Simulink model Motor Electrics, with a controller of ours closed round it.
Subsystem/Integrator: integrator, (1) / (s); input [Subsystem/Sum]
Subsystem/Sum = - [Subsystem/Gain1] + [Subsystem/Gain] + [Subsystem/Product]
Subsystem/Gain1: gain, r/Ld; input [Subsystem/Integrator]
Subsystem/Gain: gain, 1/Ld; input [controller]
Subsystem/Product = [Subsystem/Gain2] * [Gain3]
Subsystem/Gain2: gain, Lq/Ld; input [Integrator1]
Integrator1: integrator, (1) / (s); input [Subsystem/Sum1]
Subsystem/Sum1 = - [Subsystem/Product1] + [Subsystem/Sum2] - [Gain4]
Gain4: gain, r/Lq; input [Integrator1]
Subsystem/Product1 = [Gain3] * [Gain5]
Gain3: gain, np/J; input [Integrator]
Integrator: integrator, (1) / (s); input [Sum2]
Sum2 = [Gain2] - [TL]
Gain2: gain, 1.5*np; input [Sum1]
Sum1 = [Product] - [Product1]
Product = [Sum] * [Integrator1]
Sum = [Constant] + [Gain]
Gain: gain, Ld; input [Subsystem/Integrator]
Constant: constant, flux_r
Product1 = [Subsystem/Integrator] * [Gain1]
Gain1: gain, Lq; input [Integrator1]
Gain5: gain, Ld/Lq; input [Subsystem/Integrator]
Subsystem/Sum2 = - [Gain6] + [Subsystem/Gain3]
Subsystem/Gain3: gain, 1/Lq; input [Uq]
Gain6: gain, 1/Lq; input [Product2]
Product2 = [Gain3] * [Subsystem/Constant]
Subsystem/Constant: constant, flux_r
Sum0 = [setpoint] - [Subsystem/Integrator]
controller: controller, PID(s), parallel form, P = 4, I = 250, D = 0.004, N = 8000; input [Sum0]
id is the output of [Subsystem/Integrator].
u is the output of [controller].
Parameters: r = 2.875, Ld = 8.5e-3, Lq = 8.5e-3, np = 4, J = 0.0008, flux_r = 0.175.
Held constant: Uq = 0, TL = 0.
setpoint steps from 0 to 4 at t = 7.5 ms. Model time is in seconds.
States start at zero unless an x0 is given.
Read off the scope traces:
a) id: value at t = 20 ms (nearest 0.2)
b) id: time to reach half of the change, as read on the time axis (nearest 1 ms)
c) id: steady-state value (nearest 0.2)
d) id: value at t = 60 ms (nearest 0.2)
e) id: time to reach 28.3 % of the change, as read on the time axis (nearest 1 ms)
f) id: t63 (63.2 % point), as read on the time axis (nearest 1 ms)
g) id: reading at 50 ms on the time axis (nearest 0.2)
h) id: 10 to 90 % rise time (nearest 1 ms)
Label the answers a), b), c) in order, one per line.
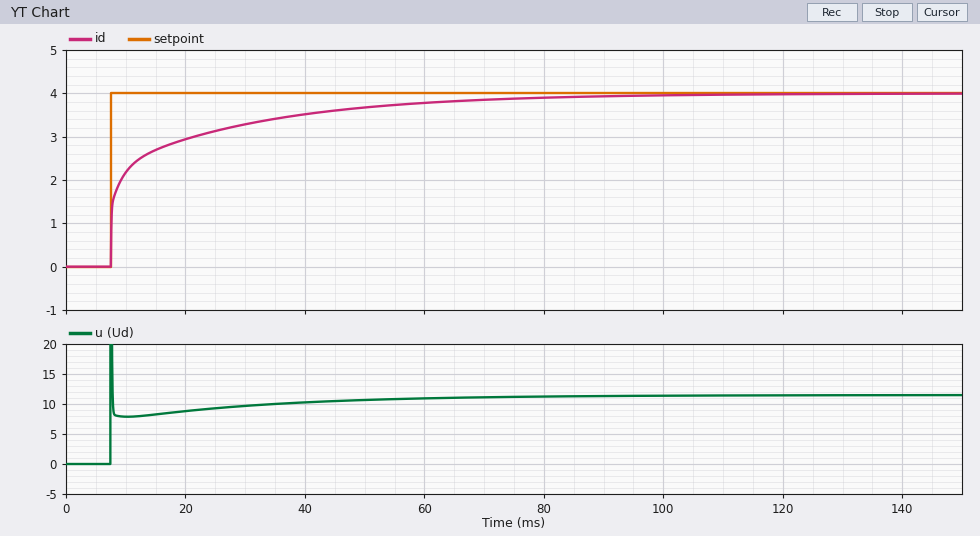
a) 3.0
b) 9 ms
c) 4.0
d) 3.8
e) 8 ms
f) 13 ms
g) 3.6
h) 37 ms
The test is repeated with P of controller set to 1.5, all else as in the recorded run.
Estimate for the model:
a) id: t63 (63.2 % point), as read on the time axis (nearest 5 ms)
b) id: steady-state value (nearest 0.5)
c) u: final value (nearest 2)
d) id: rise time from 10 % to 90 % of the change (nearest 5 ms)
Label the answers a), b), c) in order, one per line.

a) 20 ms
b) 4.0
c) 12
d) 30 ms
